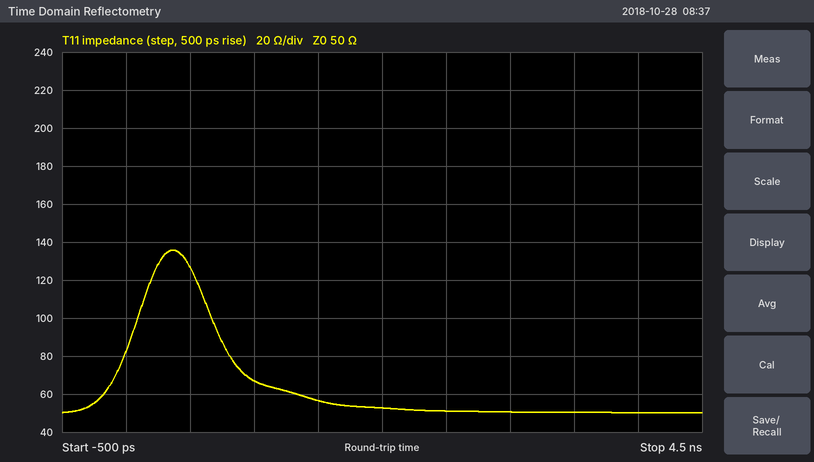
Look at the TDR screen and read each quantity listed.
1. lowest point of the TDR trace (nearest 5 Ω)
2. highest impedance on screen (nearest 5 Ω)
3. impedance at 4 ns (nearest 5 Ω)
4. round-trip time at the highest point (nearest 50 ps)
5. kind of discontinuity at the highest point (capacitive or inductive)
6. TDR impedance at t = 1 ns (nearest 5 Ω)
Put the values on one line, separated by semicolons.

50 Ω; 135 Ω; 50 Ω; 350 ps; inductive; 65 Ω
